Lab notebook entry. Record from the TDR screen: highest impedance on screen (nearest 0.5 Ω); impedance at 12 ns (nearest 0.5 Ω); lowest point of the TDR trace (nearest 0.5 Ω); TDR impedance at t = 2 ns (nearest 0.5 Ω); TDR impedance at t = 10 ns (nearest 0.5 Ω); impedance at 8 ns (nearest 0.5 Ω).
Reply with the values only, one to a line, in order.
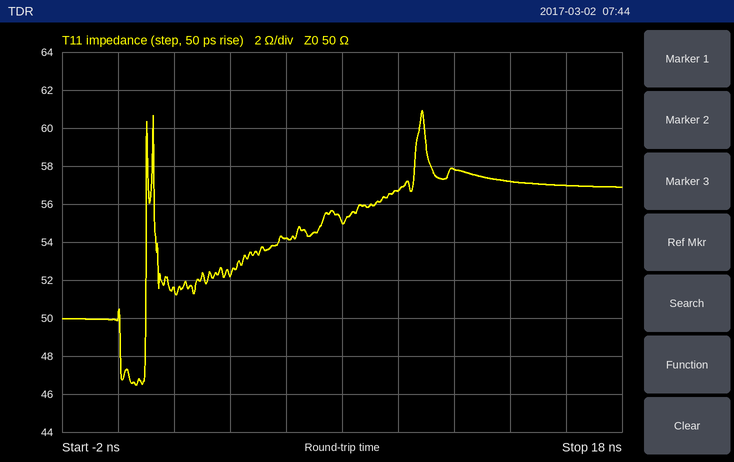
61.0 Ω
58.0 Ω
46.5 Ω
51.5 Ω
56.5 Ω
55.0 Ω
